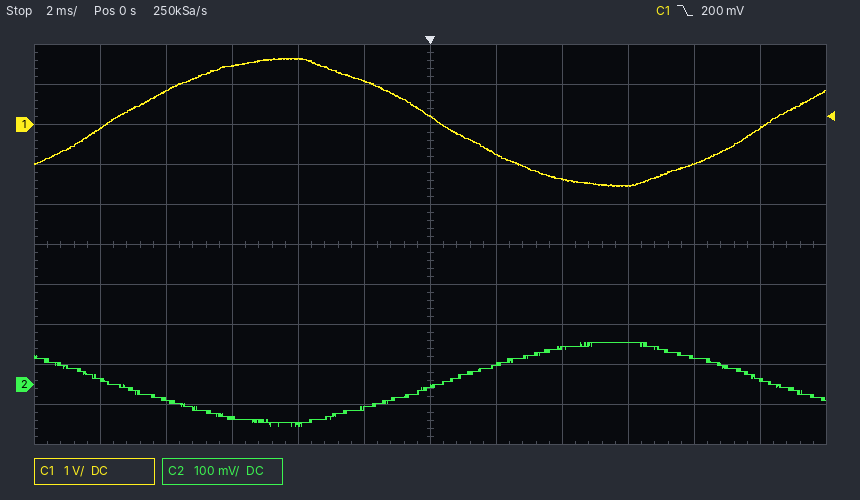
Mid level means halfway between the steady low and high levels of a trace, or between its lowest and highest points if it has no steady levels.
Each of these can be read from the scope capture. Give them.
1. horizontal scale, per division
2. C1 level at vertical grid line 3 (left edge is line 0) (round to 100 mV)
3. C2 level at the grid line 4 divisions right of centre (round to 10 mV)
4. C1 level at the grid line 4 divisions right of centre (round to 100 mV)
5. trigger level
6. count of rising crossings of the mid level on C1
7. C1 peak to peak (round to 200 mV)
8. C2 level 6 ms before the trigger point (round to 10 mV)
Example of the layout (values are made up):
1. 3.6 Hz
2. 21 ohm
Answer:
1. 2 ms
2. 1.5 V
3. 70 mV
4. -1.0 V
5. 200 mV
6. 2
7. 3.2 V
8. -80 mV
